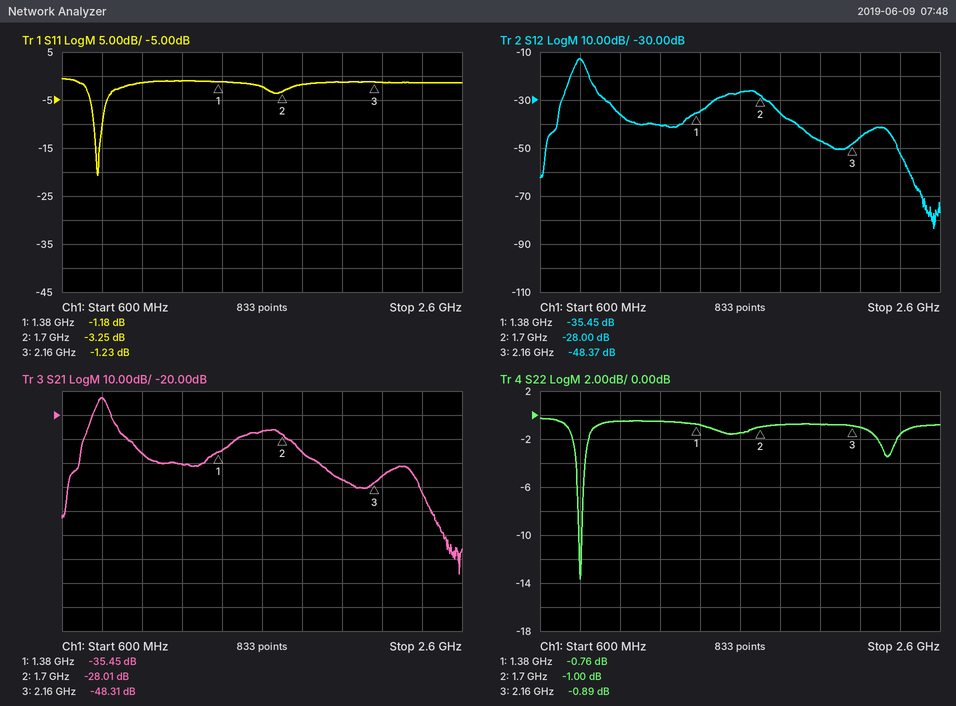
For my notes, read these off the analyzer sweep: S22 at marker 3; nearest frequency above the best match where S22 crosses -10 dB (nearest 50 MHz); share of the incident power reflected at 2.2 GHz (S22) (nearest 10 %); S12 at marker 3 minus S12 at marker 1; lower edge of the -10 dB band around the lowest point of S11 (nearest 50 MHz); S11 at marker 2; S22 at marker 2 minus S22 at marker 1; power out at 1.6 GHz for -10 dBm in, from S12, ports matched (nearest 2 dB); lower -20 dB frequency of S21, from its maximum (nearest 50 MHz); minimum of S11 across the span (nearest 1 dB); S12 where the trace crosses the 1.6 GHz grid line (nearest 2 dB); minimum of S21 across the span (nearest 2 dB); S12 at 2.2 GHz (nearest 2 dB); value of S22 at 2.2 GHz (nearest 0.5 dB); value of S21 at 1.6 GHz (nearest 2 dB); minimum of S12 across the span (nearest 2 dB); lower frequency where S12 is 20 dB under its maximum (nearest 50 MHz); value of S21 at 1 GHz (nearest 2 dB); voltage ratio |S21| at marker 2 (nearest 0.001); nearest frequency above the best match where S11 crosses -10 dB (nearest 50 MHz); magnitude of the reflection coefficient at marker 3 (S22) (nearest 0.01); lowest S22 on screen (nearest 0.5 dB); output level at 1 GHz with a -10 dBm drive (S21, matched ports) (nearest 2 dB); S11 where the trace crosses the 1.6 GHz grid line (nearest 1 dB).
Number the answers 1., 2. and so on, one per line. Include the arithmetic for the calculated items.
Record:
1. -0.89 dB
2. 800 MHz
3. 10^(-1/10) ≈ 79.4 %, so 80 % to the nearest 10 %
4. -48.37 − (-35.45) = -12.92 dB
5. 750 MHz
6. -3.25 dB
7. -1 − (-0.76) = -0.24 dB
8. -10 dBm + (-26 dB) = -36 dBm
9. 700 MHz
10. -21 dB
11. -26 dB
12. -86 dB
13. -46 dB
14. -1.0 dB
15. -26 dB
16. -84 dB
17. 700 MHz
18. -36 dB
19. 10^(-28.01/20) ≈ 0.040
20. 800 MHz
21. 10^(-0.89/20) ≈ 0.90
22. -13.5 dB
23. -10 dBm + (-36 dB) = -46 dBm
24. -2 dB
